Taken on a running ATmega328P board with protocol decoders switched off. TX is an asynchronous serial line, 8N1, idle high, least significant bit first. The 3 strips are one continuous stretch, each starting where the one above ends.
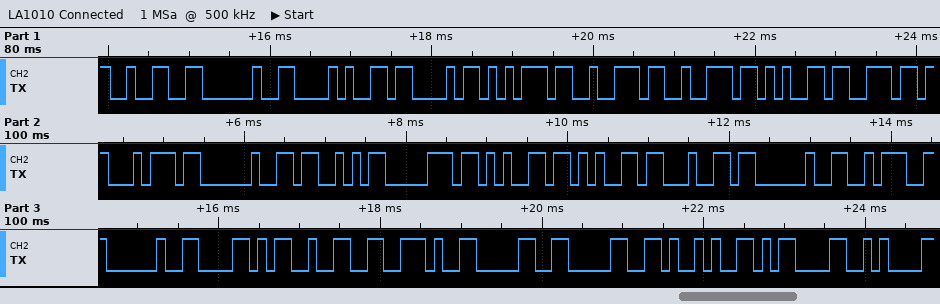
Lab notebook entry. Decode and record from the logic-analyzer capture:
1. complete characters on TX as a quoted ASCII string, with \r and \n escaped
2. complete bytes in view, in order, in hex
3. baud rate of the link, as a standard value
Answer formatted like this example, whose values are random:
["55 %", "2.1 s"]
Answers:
["\"2 (Current Speed : X2.00)\\r\\n\"", "32 20 28 43 75 72 72 65 6E 74 20 53 70 65 65 64 20 3A 20 58 32 2E 30 30 29 0D 0A", "9600 baud"]
